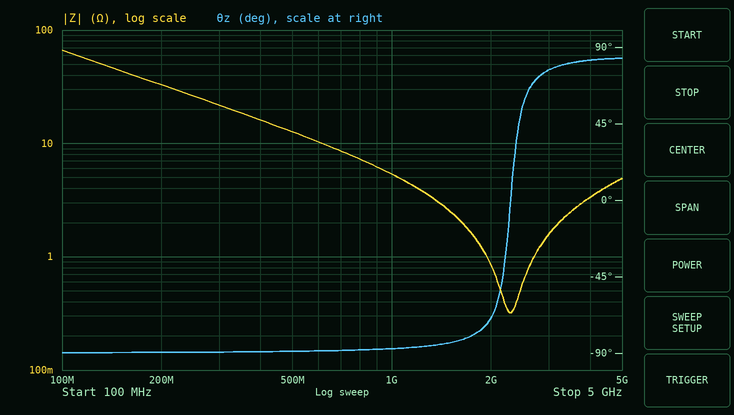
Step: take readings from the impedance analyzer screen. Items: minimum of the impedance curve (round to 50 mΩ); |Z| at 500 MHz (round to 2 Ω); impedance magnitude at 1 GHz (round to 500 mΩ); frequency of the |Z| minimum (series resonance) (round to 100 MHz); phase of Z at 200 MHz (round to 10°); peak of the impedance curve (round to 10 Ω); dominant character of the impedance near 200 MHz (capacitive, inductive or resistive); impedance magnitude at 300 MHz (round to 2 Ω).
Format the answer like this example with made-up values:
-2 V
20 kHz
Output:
300 mΩ
12 Ω
5.5 Ω
2.3 GHz
-90°
70 Ω
capacitive
22 Ω
